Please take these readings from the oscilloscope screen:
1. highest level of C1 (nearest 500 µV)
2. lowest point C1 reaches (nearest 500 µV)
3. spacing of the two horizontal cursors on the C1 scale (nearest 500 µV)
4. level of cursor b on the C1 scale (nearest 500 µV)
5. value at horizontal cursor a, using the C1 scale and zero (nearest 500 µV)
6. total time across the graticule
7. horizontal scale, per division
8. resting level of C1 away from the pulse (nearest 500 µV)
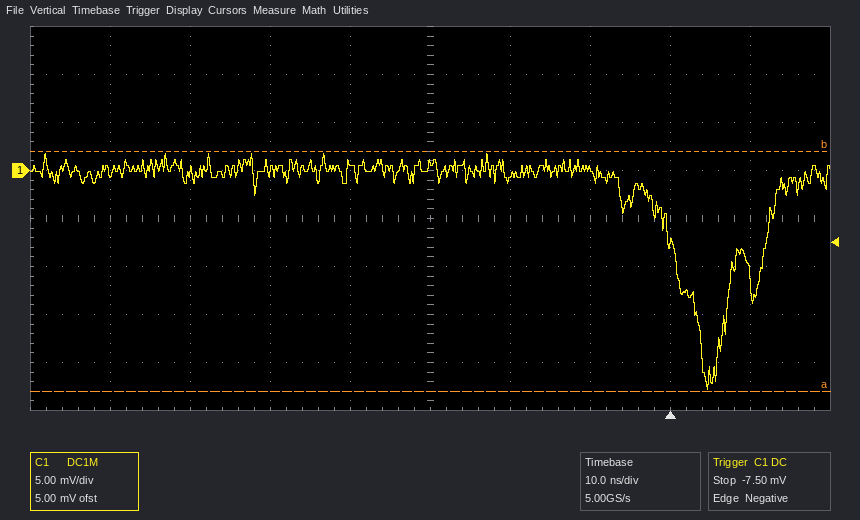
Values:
2.0 mV
-23.0 mV
25.0 mV
2.0 mV
-23.0 mV
100 ns
10 ns
0.0 mV
